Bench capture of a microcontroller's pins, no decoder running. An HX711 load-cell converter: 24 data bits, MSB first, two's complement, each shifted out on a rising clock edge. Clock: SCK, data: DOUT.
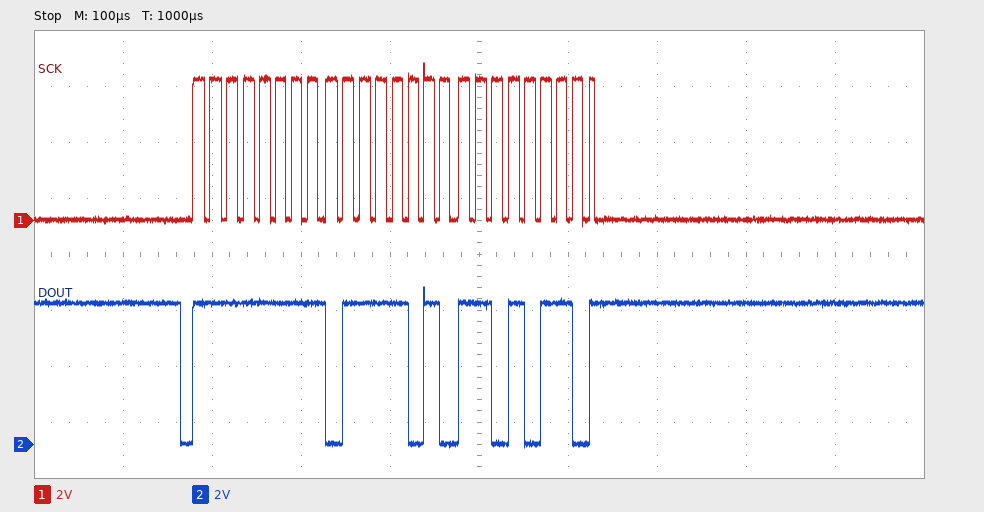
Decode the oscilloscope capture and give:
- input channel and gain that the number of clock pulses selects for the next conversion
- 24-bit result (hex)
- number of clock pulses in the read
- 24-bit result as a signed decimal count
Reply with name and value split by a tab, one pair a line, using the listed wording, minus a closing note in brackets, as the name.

input channel and gain that the number of clock pulses selects for the next conversion	channel A, gain 128
24-bit result	0xFF7AD6
number of clock pulses in the read	25
24-bit result as a signed decimal count	-34090
